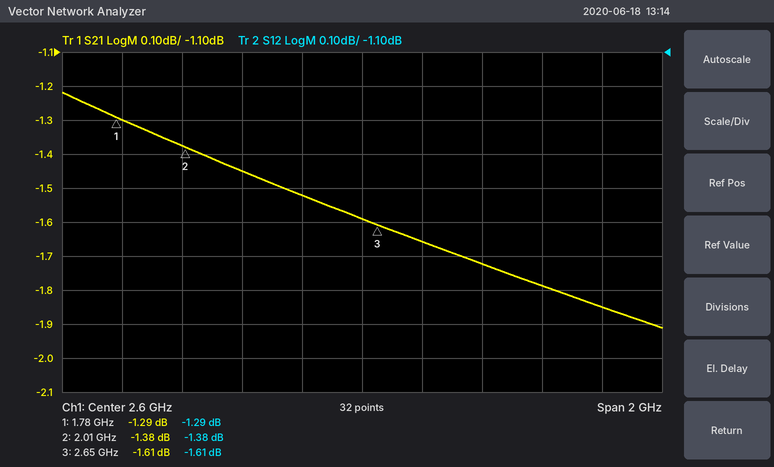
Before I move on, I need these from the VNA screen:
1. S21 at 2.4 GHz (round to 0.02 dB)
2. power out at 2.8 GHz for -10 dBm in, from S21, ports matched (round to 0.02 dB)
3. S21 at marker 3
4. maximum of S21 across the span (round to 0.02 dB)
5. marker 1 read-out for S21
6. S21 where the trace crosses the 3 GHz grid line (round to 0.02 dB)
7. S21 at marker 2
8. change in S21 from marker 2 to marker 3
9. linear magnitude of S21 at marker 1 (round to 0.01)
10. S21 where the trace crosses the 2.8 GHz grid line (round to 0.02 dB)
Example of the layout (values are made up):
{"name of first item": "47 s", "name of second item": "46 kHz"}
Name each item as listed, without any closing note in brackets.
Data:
{"S21 at 2.4 GHz": "-1.52 dB", "power out at 2.8 GHz for -10 dBm in, from S21, ports matched": "-11.66 dBm", "S21 at marker 3": "-1.61 dB", "maximum of S21 across the span": "-1.22 dB", "marker 1 read-out for S21": "-1.29 dB", "S21 where the trace crosses the 3 GHz grid line": "-1.72 dB", "S21 at marker 2": "-1.38 dB", "change in S21 from marker 2 to marker 3": "-0.23 dB", "linear magnitude of S21 at marker 1": "0.86", "S21 where the trace crosses the 2.8 GHz grid line": "-1.66 dB"}
